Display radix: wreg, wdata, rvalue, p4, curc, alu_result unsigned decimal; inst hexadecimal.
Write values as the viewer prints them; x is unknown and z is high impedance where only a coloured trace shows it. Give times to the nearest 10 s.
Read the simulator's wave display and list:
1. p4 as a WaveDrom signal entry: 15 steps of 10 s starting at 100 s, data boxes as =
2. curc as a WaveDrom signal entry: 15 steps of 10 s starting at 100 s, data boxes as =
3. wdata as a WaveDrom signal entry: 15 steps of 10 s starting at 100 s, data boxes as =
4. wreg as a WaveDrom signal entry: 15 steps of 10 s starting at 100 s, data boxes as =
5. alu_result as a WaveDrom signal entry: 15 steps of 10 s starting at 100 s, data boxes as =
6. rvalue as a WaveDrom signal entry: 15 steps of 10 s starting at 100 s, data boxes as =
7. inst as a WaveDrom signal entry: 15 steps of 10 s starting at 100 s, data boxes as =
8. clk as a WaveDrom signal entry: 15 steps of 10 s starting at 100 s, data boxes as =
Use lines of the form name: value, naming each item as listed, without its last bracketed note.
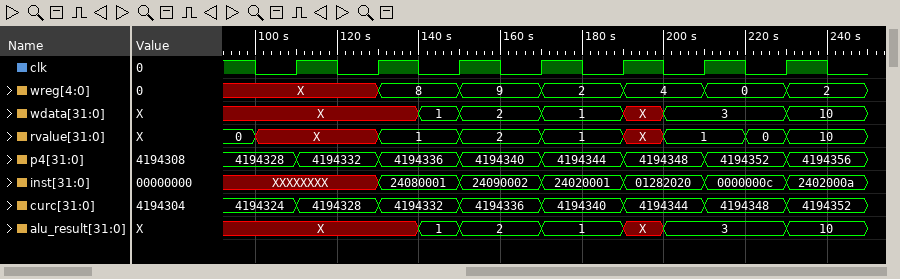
p4 as a WaveDrom signal entry: 15 steps of 10 s starting at 100 s, data boxes as =: {name: 'p4', wave: '==.=.=.=.=.=.=.', data: '4194328 4194332 4194336 4194340 4194344 4194348 4194352 4194356'}
curc as a WaveDrom signal entry: 15 steps of 10 s starting at 100 s, data boxes as =: {name: 'curc', wave: '==.=.=.=.=.=.=.', data: '4194324 4194328 4194332 4194336 4194340 4194344 4194348 4194352'}
wdata as a WaveDrom signal entry: 15 steps of 10 s starting at 100 s, data boxes as =: {name: 'wdata', wave: 'x...==.=.x=..=.', data: '1 2 1 3 10'}
wreg as a WaveDrom signal entry: 15 steps of 10 s starting at 100 s, data boxes as =: {name: 'wreg', wave: 'x..=.=.=.=.=.=.', data: '8 9 2 4 0 2'}
alu_result as a WaveDrom signal entry: 15 steps of 10 s starting at 100 s, data boxes as =: {name: 'alu_result', wave: 'x...==.=.x=..=.', data: '1 2 1 3 10'}
rvalue as a WaveDrom signal entry: 15 steps of 10 s starting at 100 s, data boxes as =: {name: 'rvalue', wave: 'x..=.=.=.x=.==.', data: '1 2 1 1 0 10'}
inst as a WaveDrom signal entry: 15 steps of 10 s starting at 100 s, data boxes as =: {name: 'inst', wave: 'x..=.=.=.=.=.=.', data: '24080001 24090002 24020001 01282020 0000000c 2402000a'}
clk as a WaveDrom signal entry: 15 steps of 10 s starting at 100 s, data boxes as =: {name: 'clk', wave: '010101010101010'}
